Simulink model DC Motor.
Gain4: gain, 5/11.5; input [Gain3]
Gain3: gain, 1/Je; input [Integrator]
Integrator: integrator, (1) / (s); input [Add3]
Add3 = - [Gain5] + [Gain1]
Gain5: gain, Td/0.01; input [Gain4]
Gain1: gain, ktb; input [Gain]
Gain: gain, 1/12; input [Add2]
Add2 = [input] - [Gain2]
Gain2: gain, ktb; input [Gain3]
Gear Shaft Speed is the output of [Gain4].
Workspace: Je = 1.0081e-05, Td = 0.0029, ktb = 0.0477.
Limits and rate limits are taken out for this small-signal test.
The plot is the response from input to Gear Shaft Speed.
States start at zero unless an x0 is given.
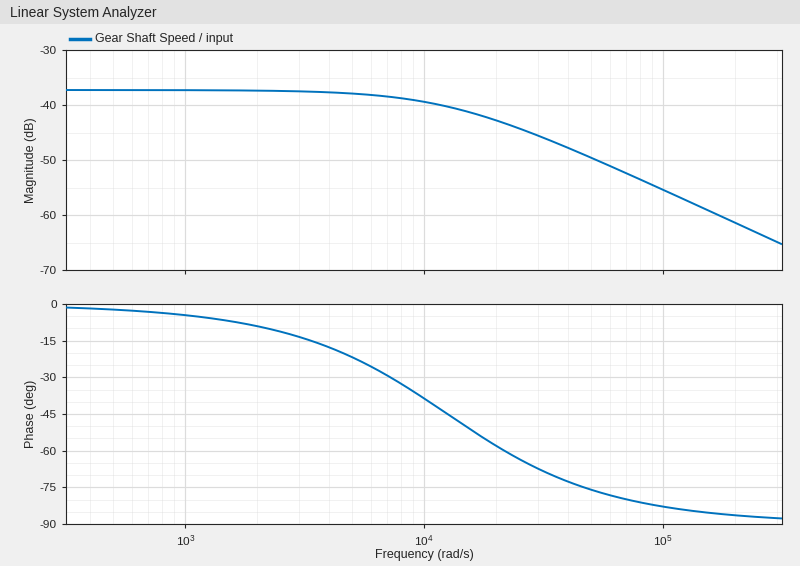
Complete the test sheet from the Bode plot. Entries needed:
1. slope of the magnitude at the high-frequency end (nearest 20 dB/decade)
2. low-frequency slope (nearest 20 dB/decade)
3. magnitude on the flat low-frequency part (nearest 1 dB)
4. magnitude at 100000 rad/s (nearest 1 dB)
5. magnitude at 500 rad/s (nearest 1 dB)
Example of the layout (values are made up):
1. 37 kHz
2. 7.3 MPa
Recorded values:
1. -20 dB/decade
2. 0 dB/decade
3. -37 dB
4. -55 dB
5. -37 dB
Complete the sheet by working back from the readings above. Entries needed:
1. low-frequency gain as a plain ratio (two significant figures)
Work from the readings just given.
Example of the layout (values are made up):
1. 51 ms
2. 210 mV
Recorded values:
1. 0.014
